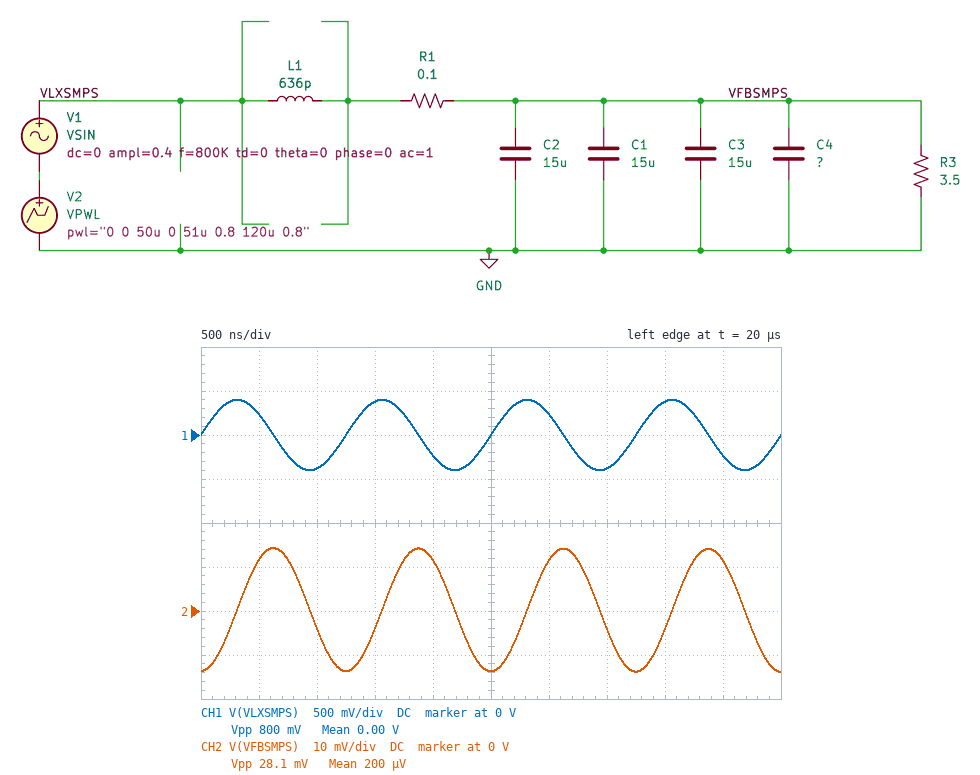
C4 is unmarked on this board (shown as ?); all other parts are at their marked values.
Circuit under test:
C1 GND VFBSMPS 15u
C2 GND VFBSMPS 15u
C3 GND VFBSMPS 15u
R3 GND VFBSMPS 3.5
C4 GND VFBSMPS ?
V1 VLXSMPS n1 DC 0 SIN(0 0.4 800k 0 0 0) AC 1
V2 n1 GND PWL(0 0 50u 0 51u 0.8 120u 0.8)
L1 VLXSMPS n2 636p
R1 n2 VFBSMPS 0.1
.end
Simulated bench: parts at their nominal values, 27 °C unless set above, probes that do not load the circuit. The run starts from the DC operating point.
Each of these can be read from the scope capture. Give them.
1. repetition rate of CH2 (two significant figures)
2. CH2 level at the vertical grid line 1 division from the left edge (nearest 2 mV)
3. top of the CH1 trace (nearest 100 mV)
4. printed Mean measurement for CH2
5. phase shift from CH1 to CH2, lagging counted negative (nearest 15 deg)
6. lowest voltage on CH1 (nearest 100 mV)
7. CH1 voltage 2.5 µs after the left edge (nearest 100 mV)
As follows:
800 kHz
12 mV
400 mV
200 µV
-90 deg
-400 mV
0 V
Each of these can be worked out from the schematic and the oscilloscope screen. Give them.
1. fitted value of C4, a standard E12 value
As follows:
12 µF
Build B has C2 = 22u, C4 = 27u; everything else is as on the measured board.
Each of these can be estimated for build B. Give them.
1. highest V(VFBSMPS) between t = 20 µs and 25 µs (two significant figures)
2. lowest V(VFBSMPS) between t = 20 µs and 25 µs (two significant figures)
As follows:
11 mV
-9.7 mV
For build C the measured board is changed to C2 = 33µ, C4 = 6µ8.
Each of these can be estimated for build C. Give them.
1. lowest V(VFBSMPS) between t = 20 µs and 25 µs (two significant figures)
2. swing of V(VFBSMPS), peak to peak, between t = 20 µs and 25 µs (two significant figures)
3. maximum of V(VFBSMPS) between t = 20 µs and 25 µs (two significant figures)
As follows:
-11 mV
23 mV
12 mV
